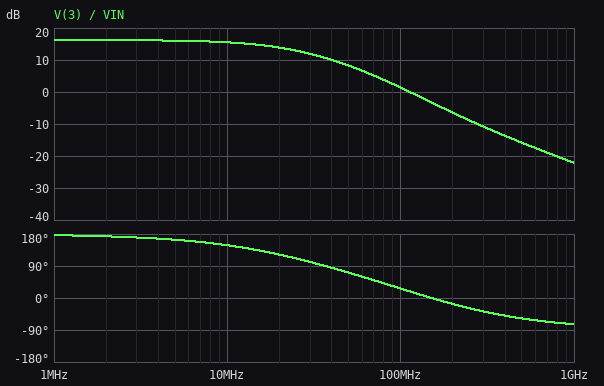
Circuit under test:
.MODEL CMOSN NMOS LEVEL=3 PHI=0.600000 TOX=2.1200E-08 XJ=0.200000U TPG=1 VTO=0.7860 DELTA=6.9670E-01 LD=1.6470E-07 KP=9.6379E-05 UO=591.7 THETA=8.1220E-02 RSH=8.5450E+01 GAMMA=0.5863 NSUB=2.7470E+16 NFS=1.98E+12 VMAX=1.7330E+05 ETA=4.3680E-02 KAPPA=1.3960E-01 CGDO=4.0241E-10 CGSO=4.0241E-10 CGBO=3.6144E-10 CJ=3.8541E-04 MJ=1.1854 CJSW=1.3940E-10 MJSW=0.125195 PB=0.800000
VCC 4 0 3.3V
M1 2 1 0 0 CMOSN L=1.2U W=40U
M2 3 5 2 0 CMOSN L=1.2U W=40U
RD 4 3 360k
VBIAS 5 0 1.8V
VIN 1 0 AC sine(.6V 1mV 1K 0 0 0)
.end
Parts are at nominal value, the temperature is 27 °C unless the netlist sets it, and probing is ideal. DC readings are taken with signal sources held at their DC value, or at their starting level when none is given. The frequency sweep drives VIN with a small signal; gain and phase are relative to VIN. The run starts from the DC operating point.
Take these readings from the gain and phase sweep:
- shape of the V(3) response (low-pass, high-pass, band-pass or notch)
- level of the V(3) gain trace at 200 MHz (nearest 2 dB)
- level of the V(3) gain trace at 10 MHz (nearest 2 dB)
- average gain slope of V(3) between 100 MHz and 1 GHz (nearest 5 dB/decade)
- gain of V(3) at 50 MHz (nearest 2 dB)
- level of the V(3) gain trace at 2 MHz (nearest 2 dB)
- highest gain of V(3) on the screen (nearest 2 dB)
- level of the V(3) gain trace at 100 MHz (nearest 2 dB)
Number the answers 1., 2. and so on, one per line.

1. low-pass
2. -6 dB
3. 16 dB
4. -25 dB/decade
5. 8 dB
6. 16 dB
7. 16 dB
8. 2 dB
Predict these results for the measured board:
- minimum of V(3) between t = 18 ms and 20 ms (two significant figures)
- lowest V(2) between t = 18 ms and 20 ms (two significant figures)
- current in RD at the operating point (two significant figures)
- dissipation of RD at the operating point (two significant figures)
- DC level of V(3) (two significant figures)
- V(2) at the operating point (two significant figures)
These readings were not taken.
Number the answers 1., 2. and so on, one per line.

1. 2.7 V
2. 1.0 V
3. 1.6 µA
4. 900 nW
5. 2.7 V
6. 1.0 V
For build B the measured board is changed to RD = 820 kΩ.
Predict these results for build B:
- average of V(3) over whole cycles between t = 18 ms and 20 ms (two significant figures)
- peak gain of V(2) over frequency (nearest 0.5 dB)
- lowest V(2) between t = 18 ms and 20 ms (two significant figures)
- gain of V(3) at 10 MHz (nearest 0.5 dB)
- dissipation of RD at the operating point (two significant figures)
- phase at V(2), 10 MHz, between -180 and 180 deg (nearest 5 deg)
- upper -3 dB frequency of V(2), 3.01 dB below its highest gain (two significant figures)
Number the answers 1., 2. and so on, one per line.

1. 2.0 V
2. 1.5 dB
3. 980 mV
4. 20.5 dB
5. 2.0 µW
6. 155 deg
7. 20 MHz
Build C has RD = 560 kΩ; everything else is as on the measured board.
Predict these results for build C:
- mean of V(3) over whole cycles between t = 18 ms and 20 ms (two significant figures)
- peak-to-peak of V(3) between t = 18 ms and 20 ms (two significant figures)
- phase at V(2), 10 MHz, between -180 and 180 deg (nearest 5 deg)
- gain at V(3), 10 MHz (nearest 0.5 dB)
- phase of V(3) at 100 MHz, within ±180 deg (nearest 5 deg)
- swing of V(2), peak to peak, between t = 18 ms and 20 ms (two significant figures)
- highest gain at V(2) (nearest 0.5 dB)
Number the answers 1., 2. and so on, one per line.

1. 2.4 V
2. 20 mV
3. 160 deg
4. 18.5 dB
5. 20 deg
6. 2.1 mV
7. 0.5 dB
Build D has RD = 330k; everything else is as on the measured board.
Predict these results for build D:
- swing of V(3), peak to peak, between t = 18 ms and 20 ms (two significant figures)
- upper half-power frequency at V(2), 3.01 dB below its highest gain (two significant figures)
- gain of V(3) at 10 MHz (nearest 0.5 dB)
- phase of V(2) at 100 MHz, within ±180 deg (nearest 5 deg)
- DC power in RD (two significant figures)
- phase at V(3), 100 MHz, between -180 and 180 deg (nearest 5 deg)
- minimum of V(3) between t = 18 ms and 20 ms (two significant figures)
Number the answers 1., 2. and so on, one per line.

1. 12 mV
2. 54 MHz
3. 15.0 dB
4. 100 deg
5. 830 nW
6. 30 deg
7. 2.8 V
